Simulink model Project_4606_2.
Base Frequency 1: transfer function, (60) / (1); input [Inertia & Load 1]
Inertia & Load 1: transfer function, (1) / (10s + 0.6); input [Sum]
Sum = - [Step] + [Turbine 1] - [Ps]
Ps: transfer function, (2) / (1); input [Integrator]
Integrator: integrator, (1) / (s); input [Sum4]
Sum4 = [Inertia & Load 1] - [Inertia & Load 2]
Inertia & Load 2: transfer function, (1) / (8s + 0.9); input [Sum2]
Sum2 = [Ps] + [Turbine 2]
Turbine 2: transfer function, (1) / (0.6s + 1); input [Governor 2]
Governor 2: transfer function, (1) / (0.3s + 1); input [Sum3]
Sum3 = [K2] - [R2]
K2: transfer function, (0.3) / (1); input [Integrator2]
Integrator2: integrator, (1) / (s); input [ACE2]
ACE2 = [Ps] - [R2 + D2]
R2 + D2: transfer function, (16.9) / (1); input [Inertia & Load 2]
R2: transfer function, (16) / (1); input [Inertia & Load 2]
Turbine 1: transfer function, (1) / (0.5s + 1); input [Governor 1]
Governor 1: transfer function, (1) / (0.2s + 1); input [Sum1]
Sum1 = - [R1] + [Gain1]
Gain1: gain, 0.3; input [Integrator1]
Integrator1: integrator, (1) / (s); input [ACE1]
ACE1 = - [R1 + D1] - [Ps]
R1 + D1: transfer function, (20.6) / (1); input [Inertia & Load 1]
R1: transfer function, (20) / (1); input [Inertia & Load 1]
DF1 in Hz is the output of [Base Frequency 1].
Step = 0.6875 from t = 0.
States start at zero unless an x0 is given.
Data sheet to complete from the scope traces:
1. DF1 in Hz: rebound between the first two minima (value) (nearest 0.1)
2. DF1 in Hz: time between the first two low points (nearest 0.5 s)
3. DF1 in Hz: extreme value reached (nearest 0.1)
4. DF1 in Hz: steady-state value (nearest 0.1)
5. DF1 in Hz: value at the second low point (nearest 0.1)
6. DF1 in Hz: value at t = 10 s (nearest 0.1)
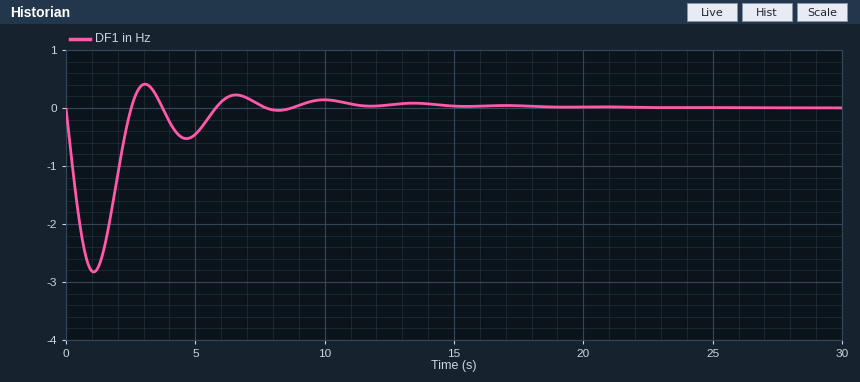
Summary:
0.4
3.5 s
-2.8
0.0
-0.5
0.1
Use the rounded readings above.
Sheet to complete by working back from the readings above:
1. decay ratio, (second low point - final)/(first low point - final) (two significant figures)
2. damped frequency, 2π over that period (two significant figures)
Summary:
0.18
1.8 rad/s
